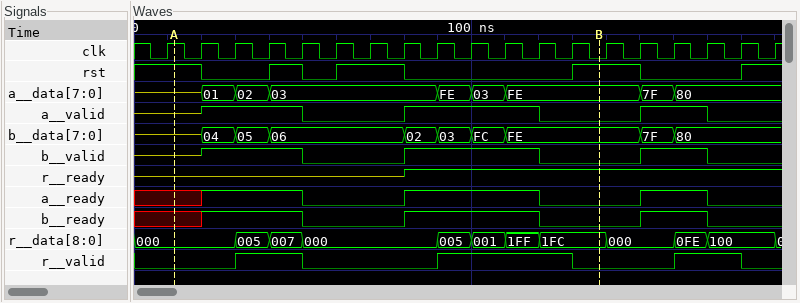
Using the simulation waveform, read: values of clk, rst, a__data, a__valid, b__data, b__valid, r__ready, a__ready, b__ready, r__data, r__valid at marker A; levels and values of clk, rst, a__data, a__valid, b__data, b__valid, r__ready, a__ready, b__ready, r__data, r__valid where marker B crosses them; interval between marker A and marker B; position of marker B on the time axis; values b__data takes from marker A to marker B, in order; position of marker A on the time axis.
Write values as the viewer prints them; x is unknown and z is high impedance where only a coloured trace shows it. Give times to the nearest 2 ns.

clk=1, rst=1, a__data=z, a__valid=z, b__data=z, b__valid=z, r__ready=z, a__ready=x, b__ready=x, r__data=000, r__valid=0
clk=0, rst=1, a__data=FE, a__valid=0, b__data=FE, b__valid=0, r__ready=1, a__ready=0, b__ready=0, r__data=1FC, r__valid=0
126 ns
138 ns
z, 04, 05, 06, 02, 03, FC, FE
12 ns
